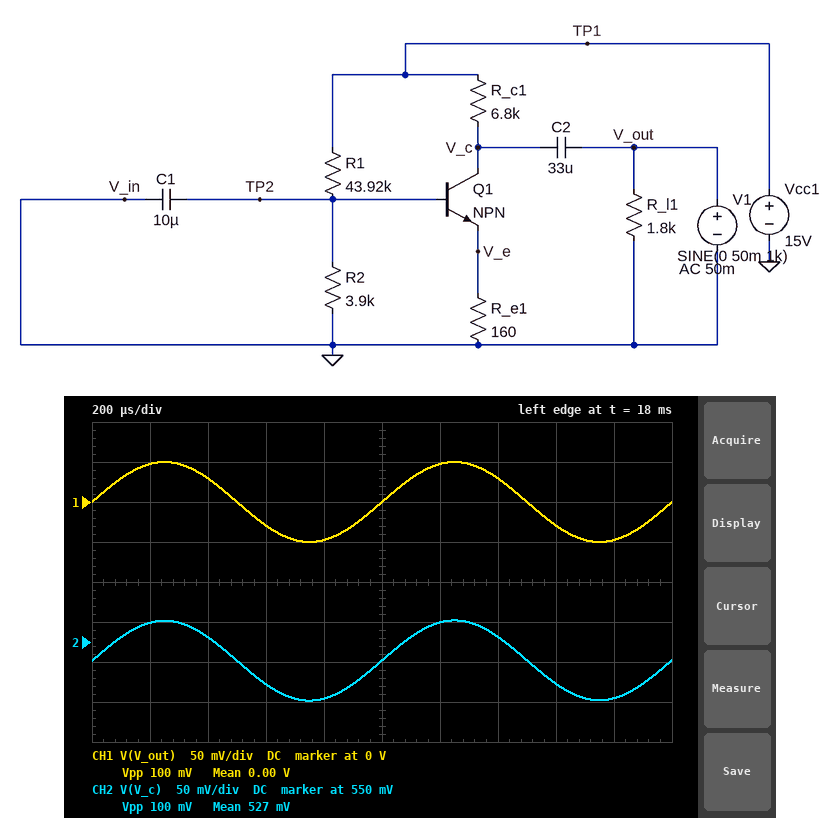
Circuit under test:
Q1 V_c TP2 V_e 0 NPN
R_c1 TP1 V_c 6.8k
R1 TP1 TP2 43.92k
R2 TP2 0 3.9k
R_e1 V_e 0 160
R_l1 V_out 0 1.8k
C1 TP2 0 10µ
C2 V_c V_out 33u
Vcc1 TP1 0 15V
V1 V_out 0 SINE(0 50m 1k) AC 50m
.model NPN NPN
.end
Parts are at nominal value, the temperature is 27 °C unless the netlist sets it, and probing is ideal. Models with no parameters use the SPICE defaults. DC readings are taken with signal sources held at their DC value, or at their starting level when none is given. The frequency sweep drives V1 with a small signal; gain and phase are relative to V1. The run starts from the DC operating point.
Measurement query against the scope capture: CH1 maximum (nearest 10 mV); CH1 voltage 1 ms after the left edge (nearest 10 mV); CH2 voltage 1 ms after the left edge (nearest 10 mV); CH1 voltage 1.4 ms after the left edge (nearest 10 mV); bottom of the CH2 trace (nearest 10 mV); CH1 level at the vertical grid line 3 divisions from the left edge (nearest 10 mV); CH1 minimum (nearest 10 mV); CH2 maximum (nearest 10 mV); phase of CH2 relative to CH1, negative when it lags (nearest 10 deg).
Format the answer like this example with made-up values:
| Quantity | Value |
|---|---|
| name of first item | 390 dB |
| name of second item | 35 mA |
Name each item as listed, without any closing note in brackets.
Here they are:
| Quantity | Value |
|---|---|
| CH1 maximum | 50 mV |
| CH1 voltage 1 ms after the left edge | 0 V |
| CH2 voltage 1 ms after the left edge | 530 mV |
| CH1 voltage 1.4 ms after the left edge | 30 mV |
| bottom of the CH2 trace | 480 mV |
| CH1 level at the vertical grid line 3 divisions from the left edge | -30 mV |
| CH1 minimum | -50 mV |
| CH2 maximum | 580 mV |
| phase of CH2 relative to CH1, negative when it lags | 0 deg |
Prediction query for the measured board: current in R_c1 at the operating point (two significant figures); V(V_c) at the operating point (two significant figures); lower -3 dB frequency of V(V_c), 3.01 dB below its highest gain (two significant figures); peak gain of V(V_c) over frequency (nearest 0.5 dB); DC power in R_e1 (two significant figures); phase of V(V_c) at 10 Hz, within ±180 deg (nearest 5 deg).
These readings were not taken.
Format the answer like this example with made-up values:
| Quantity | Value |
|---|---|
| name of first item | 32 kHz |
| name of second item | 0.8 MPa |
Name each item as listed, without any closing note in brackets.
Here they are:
| Quantity | Value |
|---|---|
| current in R_c1 at the operating point | 2.1 mA |
| V(V_c) at the operating point | 520 mV |
| lower -3 dB frequency of V(V_c), 3.01 dB below its highest gain | 5.0 Hz |
| peak gain of V(V_c) over frequency | 2.0 dB |
| DC power in R_e1 | 740 µW |
| phase of V(V_c) at 10 Hz, within ±180 deg | 25 deg |
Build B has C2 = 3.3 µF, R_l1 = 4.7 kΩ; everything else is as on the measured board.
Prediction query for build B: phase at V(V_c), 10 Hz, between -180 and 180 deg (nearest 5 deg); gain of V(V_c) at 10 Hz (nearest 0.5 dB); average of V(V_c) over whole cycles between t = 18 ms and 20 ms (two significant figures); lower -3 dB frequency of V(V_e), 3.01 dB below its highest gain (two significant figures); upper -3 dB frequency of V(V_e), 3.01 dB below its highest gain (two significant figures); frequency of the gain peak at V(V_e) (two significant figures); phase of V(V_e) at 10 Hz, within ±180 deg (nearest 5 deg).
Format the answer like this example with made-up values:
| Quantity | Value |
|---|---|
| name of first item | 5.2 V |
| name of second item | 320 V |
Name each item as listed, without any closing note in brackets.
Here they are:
| Quantity | Value |
|---|---|
| phase at V(V_c), 10 Hz, between -180 and 180 deg | 120 deg |
| gain of V(V_c) at 10 Hz | -11.0 dB |
| average of V(V_c) over whole cycles between t = 18 ms and 20 ms | 540 mV |
| lower -3 dB frequency of V(V_e), 3.01 dB below its highest gain | 15 Hz |
| upper -3 dB frequency of V(V_e), 3.01 dB below its highest gain | 33 Hz |
| frequency of the gain peak at V(V_e) | 22 Hz |
| phase of V(V_e) at 10 Hz, within ±180 deg | 65 deg |
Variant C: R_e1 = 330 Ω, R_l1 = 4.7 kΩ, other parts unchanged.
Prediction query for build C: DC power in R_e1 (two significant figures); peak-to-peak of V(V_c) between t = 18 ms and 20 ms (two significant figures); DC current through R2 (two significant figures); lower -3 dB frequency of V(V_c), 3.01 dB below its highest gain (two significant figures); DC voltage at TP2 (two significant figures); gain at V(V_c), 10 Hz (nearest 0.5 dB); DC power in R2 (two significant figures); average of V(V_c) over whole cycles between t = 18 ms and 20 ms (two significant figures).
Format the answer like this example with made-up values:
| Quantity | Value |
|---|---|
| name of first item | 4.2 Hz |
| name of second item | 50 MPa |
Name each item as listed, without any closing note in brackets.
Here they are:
| Quantity | Value |
|---|---|
| DC power in R_e1 | 490 µW |
| peak-to-peak of V(V_c) between t = 18 ms and 20 ms | 100 mV |
| DC current through R2 | 300 µA |
| lower -3 dB frequency of V(V_c), 3.01 dB below its highest gain | 710 mHz |
| DC voltage at TP2 | 1.2 V |
| gain at V(V_c), 10 Hz | 0 dB |
| DC power in R2 | 360 µW |
| average of V(V_c) over whole cycles between t = 18 ms and 20 ms | 6.8 V |
